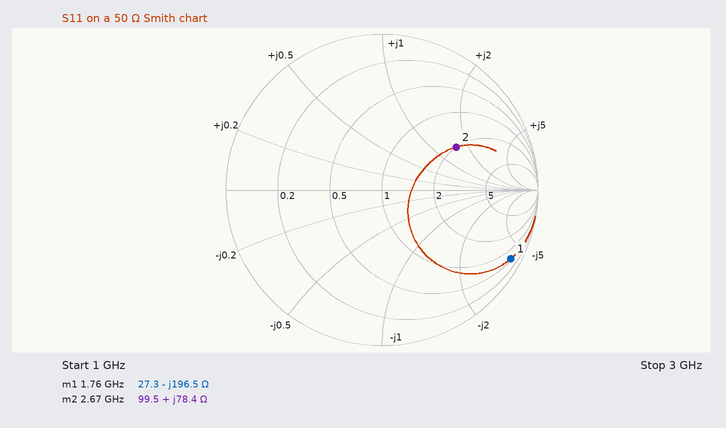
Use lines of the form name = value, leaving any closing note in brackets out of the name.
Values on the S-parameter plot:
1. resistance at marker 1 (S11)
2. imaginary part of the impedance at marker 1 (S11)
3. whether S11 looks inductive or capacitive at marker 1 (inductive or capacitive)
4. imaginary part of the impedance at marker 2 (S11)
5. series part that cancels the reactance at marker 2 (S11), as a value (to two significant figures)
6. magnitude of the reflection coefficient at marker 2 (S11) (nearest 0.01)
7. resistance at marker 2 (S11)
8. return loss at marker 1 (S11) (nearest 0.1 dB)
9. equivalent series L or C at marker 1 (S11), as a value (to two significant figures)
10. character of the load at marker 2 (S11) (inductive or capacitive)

resistance at marker 1 = 27.3 Ω
imaginary part of the impedance at marker 1 = -196.5 Ω
whether S11 looks inductive or capacitive at marker 1 = capacitive
imaginary part of the impedance at marker 2 = +78.4 Ω
series part that cancels the reactance at marker 2 (S11), as a value = 760 fF
magnitude of the reflection coefficient at marker 2 (S11) = 0.55
resistance at marker 2 = 99.5 Ω
return loss at marker 1 (S11) = 0.6 dB
equivalent series L or C at marker 1 (S11), as a value = 460 fF
character of the load at marker 2 (S11) = inductive
